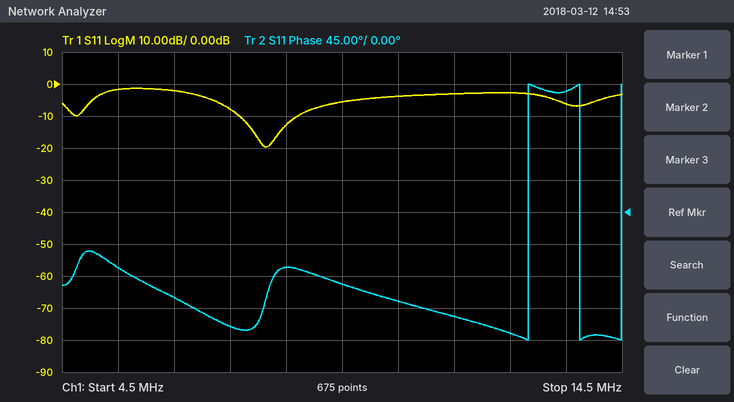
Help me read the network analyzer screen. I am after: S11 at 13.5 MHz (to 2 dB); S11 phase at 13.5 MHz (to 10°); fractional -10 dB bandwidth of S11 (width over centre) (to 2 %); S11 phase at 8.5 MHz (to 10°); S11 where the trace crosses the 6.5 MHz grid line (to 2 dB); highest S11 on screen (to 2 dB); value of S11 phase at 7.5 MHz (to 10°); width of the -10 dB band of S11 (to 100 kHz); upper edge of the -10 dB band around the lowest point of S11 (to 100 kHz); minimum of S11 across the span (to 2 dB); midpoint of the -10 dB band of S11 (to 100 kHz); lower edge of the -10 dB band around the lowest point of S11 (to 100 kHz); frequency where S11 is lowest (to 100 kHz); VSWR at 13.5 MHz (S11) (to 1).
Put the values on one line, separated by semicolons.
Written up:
-6 dB; 170°; 12 %; -80°; -2 dB; -2 dB; -160°; 1.0 MHz; 8.7 MHz; -20 dB; 8.2 MHz; 7.7 MHz; 8.1 MHz; 3
